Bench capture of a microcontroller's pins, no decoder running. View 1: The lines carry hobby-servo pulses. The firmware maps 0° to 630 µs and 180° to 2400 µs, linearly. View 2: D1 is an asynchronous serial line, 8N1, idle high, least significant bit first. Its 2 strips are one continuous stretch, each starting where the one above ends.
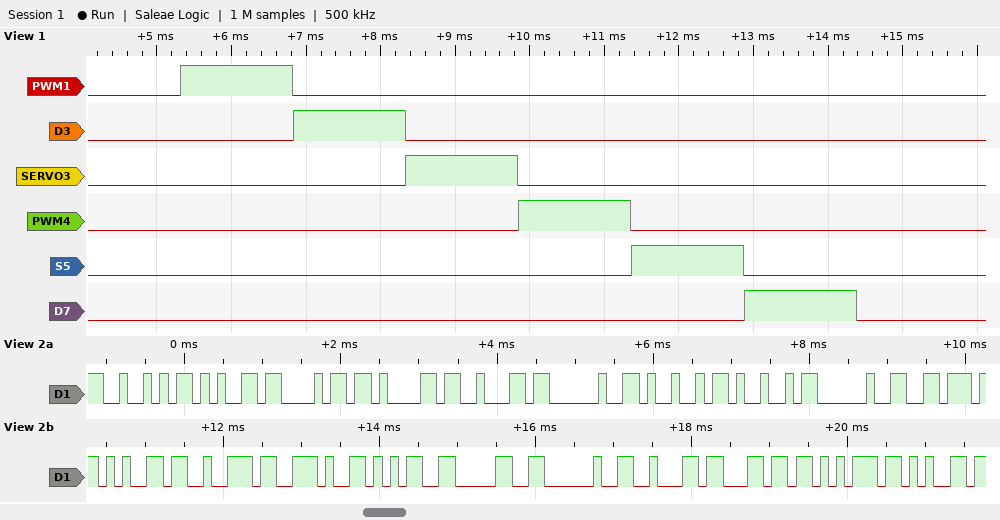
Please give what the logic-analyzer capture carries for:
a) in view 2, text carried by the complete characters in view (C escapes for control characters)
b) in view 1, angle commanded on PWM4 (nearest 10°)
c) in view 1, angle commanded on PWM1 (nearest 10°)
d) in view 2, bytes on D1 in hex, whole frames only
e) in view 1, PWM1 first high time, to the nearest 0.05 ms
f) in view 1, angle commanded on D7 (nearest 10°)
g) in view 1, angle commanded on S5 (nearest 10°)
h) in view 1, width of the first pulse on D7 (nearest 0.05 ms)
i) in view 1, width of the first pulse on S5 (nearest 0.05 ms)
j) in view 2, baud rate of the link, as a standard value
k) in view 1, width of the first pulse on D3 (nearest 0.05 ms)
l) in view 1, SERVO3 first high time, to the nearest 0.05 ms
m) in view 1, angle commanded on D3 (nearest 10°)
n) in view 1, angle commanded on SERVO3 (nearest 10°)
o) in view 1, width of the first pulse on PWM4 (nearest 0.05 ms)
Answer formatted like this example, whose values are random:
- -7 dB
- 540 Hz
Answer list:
- "Rehab II ver.50 blue"
- 90°
- 90°
- 0x52 0x65 0x68 0x61 0x62 0x20 0x49 0x49 0x20 0x76 0x65 0x72 0x2E 0x35 0x30 0x20 0x62 0x6C 0x75 0x65
- 1.50 ms
- 90°
- 90°
- 1.50 ms
- 1.50 ms
- 9600 baud
- 1.50 ms
- 1.50 ms
- 90°
- 90°
- 1.50 ms
